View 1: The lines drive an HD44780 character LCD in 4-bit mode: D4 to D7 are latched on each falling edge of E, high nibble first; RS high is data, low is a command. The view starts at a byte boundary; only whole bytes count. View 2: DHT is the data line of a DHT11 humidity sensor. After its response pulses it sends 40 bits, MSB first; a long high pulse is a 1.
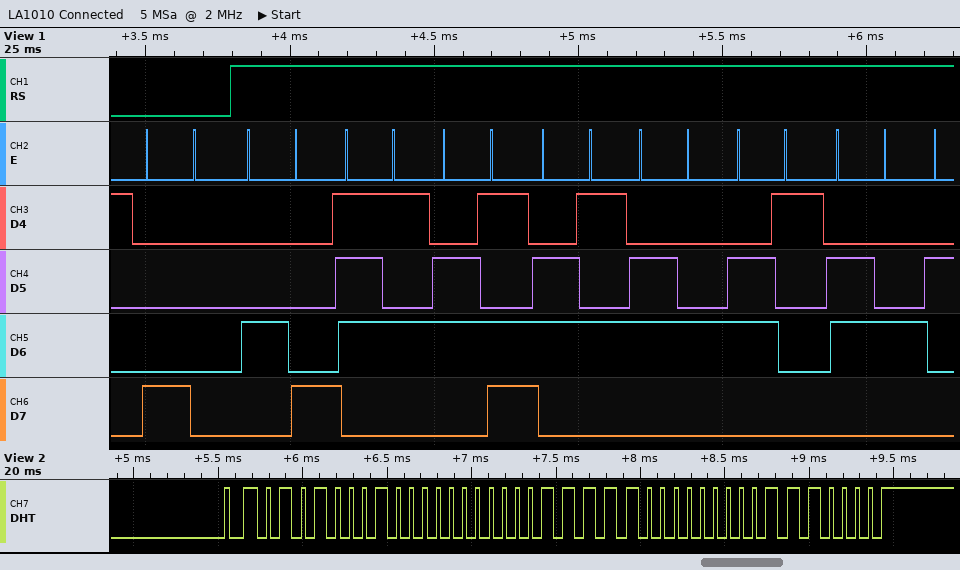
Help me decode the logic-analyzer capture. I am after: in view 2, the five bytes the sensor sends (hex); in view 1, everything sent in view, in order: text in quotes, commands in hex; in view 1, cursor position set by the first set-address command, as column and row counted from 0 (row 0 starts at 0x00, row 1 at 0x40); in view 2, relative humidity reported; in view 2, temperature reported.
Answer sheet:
51 00 1F 00 70
0x80 "Humedad"
column 0, row 0
81 %
31.0 °C
